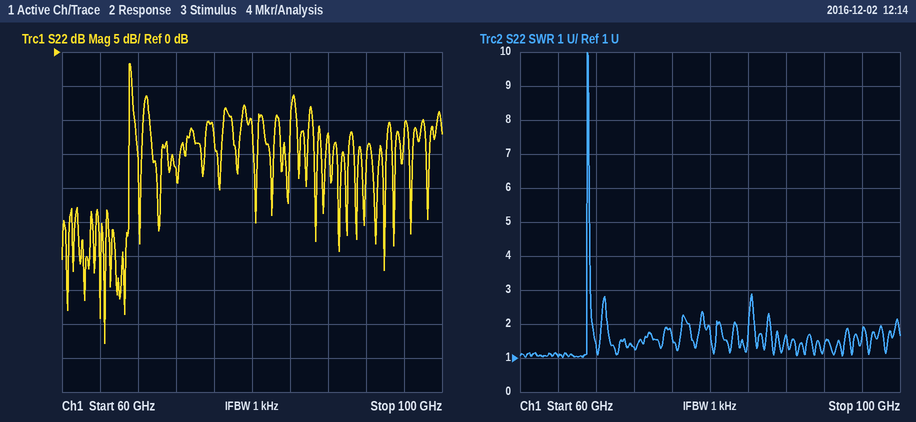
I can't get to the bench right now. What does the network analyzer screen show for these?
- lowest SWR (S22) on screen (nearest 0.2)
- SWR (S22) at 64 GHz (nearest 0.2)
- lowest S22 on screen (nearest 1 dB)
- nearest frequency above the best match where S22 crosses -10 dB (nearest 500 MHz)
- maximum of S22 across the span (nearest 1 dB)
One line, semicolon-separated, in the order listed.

1.0; 1.0; -43 dB; 67.0 GHz; -2 dB
